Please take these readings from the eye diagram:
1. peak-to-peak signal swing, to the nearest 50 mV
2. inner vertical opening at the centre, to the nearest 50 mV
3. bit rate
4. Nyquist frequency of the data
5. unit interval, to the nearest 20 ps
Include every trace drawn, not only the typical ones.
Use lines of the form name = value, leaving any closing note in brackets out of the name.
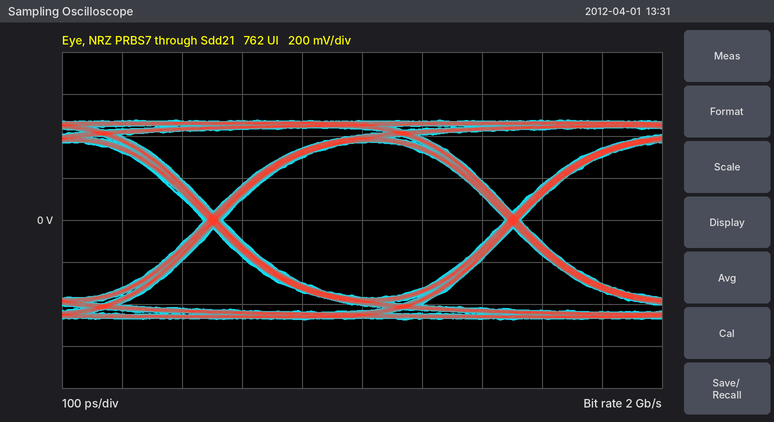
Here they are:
peak-to-peak signal swing, to the nearest 50 mV = 950 mV
inner vertical opening at the centre, to the nearest 50 mV = 750 mV
bit rate = 2 Gb/s
Nyquist frequency of the data = 1 GHz
unit interval, to the nearest 20 ps = 500 ps
